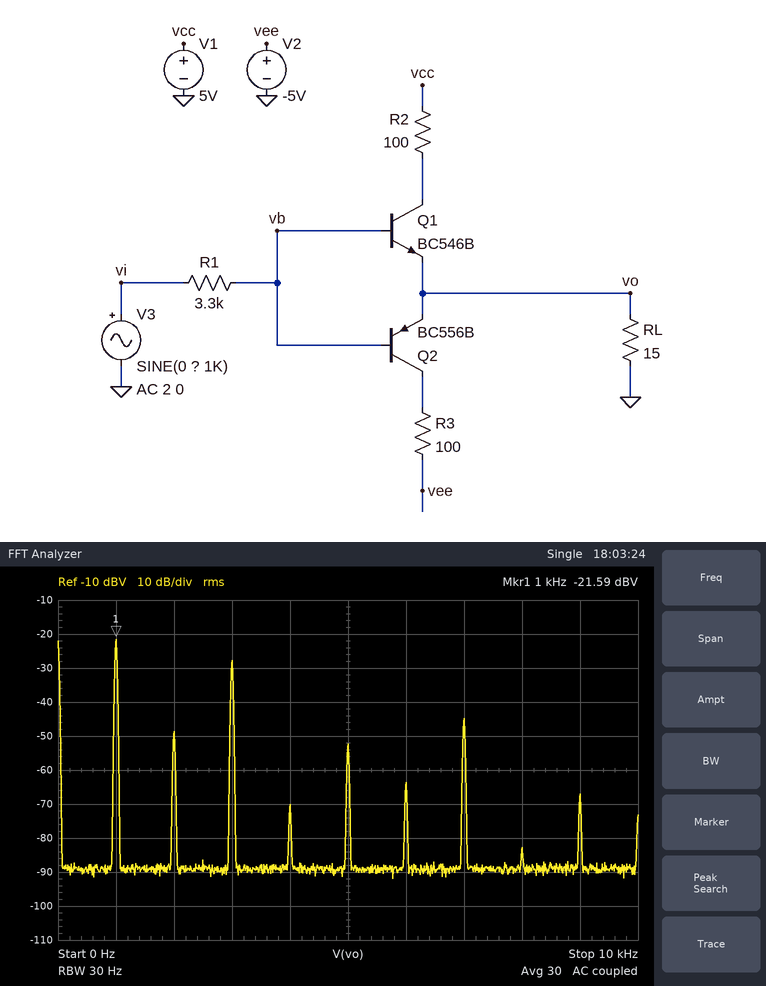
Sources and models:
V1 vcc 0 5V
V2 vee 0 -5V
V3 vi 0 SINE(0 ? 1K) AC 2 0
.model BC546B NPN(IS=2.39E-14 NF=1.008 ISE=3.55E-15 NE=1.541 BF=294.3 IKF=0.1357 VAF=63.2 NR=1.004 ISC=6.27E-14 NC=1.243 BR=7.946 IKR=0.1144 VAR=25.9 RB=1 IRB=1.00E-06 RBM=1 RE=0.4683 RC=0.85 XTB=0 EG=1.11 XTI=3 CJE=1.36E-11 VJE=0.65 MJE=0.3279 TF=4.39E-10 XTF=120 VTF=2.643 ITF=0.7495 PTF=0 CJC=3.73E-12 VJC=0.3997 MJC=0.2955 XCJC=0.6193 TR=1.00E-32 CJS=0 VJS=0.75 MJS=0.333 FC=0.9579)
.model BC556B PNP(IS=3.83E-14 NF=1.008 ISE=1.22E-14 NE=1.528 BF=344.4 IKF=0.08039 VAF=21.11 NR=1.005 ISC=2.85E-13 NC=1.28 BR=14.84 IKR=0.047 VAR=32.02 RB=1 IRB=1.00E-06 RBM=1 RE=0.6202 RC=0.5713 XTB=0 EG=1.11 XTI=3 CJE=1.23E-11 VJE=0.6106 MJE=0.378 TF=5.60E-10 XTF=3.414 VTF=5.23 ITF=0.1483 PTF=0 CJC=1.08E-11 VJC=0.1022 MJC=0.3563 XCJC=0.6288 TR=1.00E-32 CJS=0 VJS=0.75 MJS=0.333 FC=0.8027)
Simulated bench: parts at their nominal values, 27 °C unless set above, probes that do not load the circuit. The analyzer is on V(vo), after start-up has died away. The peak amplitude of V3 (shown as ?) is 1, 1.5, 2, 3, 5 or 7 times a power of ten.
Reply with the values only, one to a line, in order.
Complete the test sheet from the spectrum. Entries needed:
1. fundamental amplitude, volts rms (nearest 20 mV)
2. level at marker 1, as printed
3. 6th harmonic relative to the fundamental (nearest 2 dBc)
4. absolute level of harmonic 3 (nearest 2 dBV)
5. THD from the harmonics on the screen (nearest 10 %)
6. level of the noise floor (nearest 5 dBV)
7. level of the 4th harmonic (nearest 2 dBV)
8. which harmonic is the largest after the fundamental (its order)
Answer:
80 mV
-21.59 dBV
-42 dBc
-28 dBV
50 %
-90 dBV
-70 dBV
3
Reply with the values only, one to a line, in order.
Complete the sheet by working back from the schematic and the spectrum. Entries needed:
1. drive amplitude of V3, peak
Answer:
1 V
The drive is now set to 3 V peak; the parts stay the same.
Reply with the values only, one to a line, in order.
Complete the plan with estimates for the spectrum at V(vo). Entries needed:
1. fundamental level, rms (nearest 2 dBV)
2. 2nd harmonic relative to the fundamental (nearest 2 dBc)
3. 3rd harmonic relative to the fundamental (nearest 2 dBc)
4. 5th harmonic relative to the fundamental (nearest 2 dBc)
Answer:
-6 dBV
-50 dBc
-24 dBc
-20 dBc
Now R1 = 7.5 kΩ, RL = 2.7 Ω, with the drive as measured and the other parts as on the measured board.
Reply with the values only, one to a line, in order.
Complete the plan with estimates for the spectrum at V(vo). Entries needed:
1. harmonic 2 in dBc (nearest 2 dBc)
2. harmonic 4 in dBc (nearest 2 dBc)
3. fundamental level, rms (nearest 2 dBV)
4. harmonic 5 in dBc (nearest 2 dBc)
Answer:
-22 dBc
-40 dBc
-36 dBV
-34 dBc
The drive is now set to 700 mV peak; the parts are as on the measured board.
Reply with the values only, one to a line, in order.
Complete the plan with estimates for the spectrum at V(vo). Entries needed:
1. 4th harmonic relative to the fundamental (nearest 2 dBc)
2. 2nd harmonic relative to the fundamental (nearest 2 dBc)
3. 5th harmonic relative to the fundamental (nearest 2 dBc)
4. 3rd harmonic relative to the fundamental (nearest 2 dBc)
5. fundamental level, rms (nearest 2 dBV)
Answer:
-22 dBc
-18 dBc
-8 dBc
-2 dBc
-40 dBV
